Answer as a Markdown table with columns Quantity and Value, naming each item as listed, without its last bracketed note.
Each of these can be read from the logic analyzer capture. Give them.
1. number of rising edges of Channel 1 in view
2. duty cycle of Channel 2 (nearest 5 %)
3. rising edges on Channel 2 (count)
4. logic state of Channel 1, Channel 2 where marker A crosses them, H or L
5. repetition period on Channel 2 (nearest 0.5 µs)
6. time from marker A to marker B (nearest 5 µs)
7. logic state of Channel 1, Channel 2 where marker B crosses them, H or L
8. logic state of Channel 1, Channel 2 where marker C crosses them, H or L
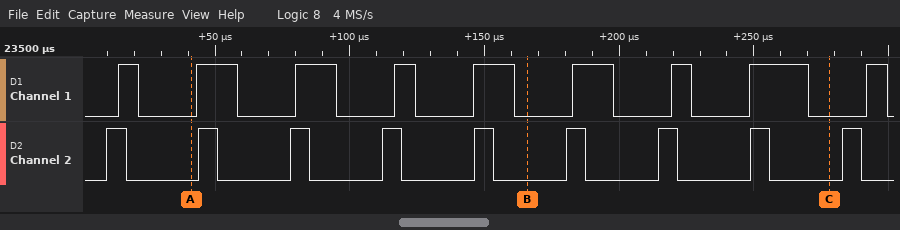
| Quantity | Value |
|---|---|
| number of rising edges of Channel 1 in view | 9 |
| duty cycle of Channel 2 | 20 % |
| rising edges on Channel 2 | 9 |
| logic state of Channel 1, Channel 2 where marker A crosses them, H or L | Channel 1=L, Channel 2=L |
| repetition period on Channel 2 | 34 µs |
| time from marker A to marker B | 125 µs |
| logic state of Channel 1, Channel 2 where marker B crosses them, H or L | Channel 1=L, Channel 2=L |
| logic state of Channel 1, Channel 2 where marker C crosses them, H or L | Channel 1=L, Channel 2=L |
